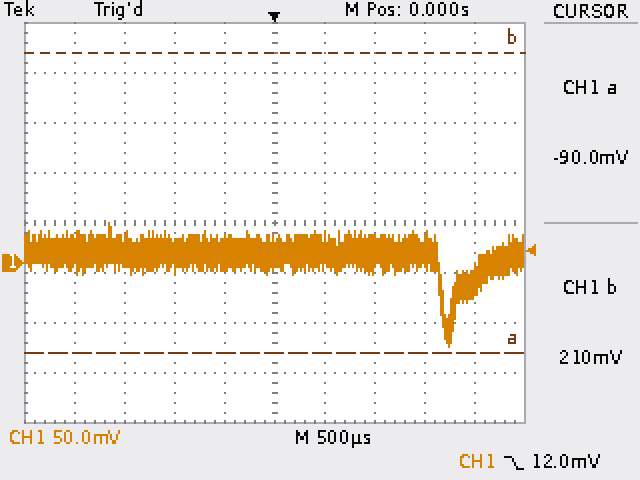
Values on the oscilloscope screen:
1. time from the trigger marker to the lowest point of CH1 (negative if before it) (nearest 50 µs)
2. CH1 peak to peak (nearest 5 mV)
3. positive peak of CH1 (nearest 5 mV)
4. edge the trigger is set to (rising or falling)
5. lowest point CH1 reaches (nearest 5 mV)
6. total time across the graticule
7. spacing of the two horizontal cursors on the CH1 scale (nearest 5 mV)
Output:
+1.75 ms
125 mV
40 mV
falling
-85 mV
5 ms
300 mV
